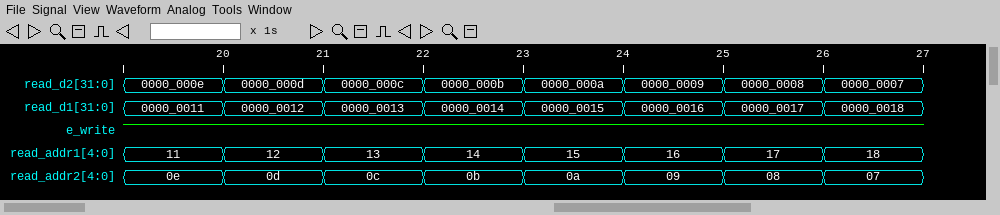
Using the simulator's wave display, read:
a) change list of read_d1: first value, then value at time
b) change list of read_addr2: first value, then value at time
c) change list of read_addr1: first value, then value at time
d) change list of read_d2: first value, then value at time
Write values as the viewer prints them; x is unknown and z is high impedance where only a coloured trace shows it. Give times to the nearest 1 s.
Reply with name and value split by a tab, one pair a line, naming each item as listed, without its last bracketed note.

change list of read_d1: first value, then value at time	0000_0011, 0000_0012 at 20 s, 0000_0013 at 21 s, 0000_0014 at 22 s, 0000_0015 at 23 s, 0000_0016 at 24 s, 0000_0017 at 25 s, 0000_0018 at 26 s
change list of read_addr2: first value, then value at time	0e, 0d at 20 s, 0c at 21 s, 0b at 22 s, 0a at 23 s, 09 at 24 s, 08 at 25 s, 07 at 26 s
change list of read_addr1: first value, then value at time	11, 12 at 20 s, 13 at 21 s, 14 at 22 s, 15 at 23 s, 16 at 24 s, 17 at 25 s, 18 at 26 s
change list of read_d2: first value, then value at time	0000_000e, 0000_000d at 20 s, 0000_000c at 21 s, 0000_000b at 22 s, 0000_000a at 23 s, 0000_0009 at 24 s, 0000_0008 at 25 s, 0000_0007 at 26 s
